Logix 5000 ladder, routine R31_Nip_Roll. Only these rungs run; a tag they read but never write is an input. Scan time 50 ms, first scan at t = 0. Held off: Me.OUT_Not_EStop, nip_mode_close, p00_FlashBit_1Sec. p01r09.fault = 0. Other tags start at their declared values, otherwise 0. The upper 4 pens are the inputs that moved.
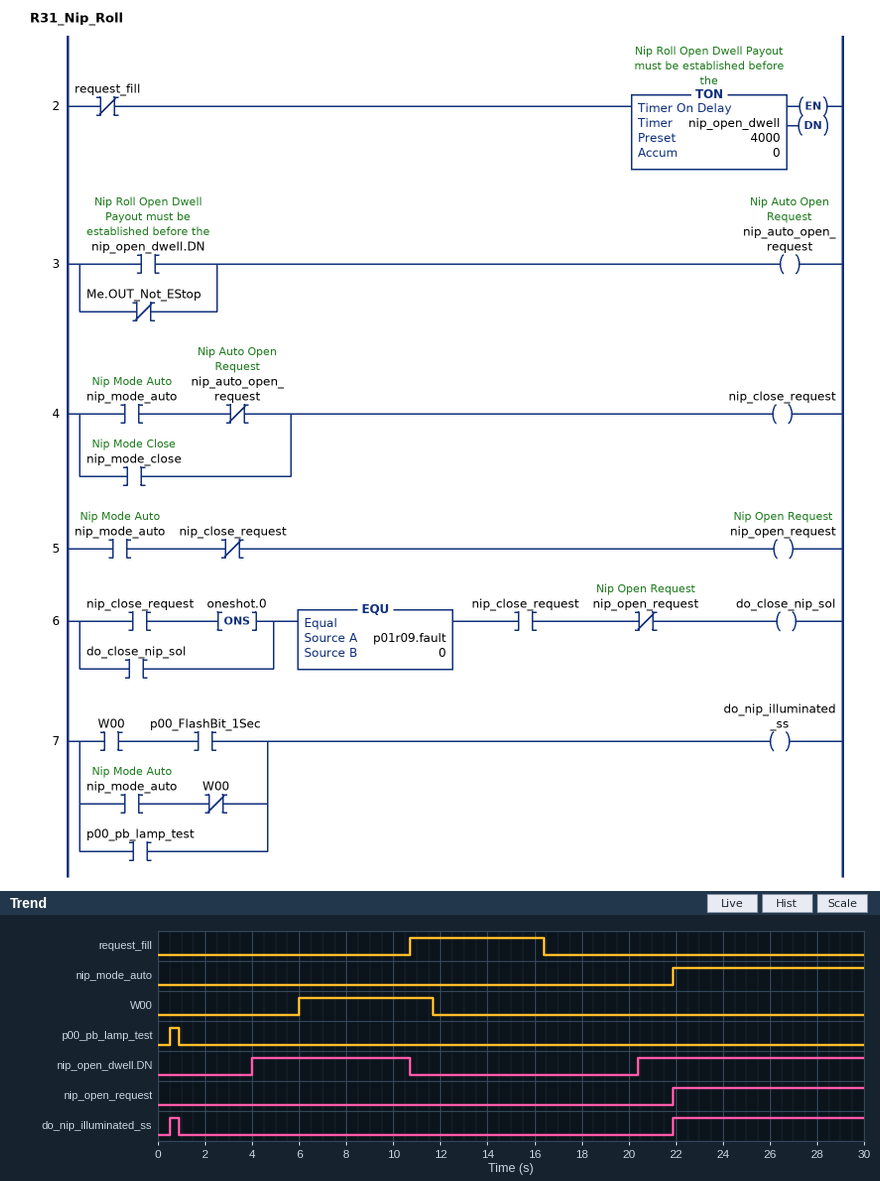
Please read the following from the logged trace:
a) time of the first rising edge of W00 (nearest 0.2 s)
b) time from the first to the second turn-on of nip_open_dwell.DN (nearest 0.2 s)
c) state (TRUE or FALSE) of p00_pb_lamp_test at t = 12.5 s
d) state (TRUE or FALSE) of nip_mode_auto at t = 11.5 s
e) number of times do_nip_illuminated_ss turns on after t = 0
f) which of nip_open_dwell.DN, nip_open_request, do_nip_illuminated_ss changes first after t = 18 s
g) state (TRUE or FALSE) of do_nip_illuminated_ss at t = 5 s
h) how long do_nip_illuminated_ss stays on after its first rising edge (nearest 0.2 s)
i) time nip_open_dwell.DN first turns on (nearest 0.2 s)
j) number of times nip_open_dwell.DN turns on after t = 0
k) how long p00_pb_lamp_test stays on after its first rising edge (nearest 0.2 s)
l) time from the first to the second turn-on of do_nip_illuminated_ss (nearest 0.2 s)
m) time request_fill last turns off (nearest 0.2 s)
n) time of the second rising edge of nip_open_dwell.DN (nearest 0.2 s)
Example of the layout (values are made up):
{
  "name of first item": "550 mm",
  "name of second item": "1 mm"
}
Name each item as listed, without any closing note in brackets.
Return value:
{
  "time of the first rising edge of W00": "6.0 s",
  "time from the first to the second turn-on of nip_open_dwell.DN": "16.4 s",
  "state (TRUE or FALSE) of p00_pb_lamp_test at t = 12.5 s": "FALSE",
  "state (TRUE or FALSE) of nip_mode_auto at t = 11.5 s": "FALSE",
  "number of times do_nip_illuminated_ss turns on after t = 0": "2",
  "which of nip_open_dwell.DN, nip_open_request, do_nip_illuminated_ss changes first after t = 18 s": "nip_open_dwell.DN",
  "state (TRUE or FALSE) of do_nip_illuminated_ss at t = 5 s": "FALSE",
  "how long do_nip_illuminated_ss stays on after its first rising edge": "0.4 s",
  "time nip_open_dwell.DN first turns on": "4.0 s",
  "number of times nip_open_dwell.DN turns on after t = 0": "2",
  "how long p00_pb_lamp_test stays on after its first rising edge": "0.4 s",
  "time from the first to the second turn-on of do_nip_illuminated_ss": "21.4 s",
  "time request_fill last turns off": "16.4 s",
  "time of the second rising edge of nip_open_dwell.DN": "20.4 s"
}
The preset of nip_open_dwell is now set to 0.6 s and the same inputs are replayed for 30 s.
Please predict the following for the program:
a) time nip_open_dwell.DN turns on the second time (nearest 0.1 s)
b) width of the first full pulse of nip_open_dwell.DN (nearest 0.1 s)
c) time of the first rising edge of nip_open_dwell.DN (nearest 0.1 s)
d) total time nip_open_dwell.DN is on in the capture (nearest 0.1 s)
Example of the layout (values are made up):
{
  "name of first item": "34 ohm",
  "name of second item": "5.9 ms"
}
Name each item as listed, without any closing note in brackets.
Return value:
{
  "time nip_open_dwell.DN turns on the second time": "17.0 s",
  "width of the first full pulse of nip_open_dwell.DN": "10.1 s",
  "time of the first rising edge of nip_open_dwell.DN": "0.6 s",
  "total time nip_open_dwell.DN is on in the capture": "23.1 s"
}
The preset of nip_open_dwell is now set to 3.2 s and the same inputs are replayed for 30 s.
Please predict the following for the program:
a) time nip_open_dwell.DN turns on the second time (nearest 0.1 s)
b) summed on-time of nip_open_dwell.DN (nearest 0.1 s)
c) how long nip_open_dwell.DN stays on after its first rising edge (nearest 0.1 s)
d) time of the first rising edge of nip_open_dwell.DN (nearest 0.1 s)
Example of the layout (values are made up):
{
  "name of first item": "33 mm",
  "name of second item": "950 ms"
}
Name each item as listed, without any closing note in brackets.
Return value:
{
  "time nip_open_dwell.DN turns on the second time": "19.6 s",
  "summed on-time of nip_open_dwell.DN": "17.9 s",
  "how long nip_open_dwell.DN stays on after its first rising edge": "7.5 s",
  "time of the first rising edge of nip_open_dwell.DN": "3.2 s"
}
